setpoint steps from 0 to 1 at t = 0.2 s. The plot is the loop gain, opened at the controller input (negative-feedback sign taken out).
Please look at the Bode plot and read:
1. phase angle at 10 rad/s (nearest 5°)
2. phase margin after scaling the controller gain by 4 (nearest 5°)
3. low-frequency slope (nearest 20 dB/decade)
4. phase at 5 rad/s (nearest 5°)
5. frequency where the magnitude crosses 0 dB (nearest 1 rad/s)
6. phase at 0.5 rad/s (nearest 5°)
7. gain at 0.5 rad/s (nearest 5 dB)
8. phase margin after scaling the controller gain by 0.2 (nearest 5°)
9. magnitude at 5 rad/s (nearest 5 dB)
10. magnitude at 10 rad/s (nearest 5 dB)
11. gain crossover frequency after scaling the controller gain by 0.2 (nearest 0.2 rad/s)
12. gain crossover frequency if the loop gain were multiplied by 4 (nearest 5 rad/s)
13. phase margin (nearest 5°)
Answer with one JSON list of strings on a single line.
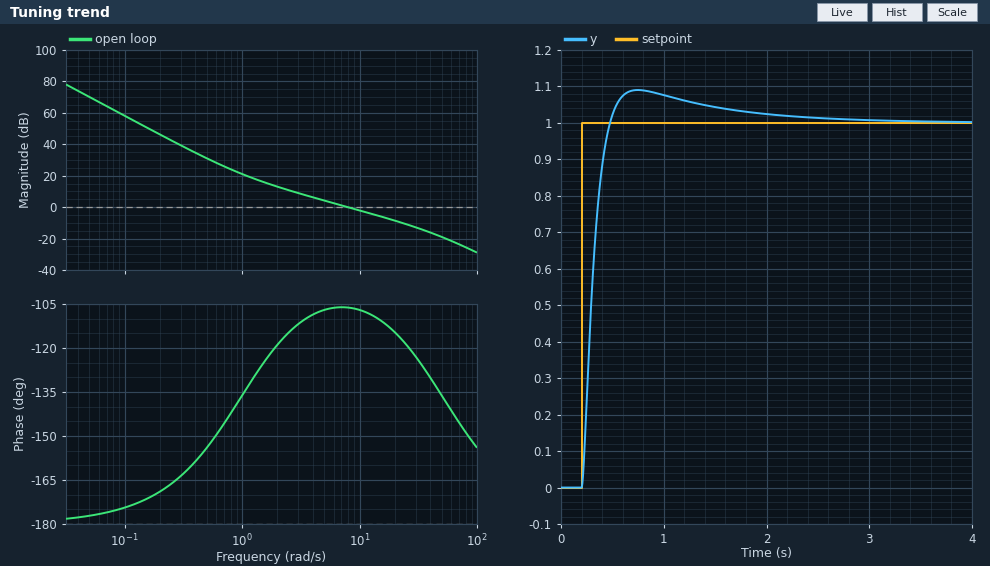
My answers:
["-105°", "60°", "-40 dB/decade", "-105°", "8 rad/s", "-155°", "30 dB", "60°", "5 dB", "0 dB", "1.8 rad/s", "30 rad/s", "75°"]
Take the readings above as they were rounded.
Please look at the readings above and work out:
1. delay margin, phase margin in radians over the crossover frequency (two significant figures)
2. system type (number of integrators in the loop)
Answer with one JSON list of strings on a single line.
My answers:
["0.16 s", "2"]
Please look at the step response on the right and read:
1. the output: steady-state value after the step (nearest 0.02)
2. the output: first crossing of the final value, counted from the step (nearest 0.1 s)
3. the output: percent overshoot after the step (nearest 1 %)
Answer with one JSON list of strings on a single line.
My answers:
["1.00", "0.3 s", "9 %"]
